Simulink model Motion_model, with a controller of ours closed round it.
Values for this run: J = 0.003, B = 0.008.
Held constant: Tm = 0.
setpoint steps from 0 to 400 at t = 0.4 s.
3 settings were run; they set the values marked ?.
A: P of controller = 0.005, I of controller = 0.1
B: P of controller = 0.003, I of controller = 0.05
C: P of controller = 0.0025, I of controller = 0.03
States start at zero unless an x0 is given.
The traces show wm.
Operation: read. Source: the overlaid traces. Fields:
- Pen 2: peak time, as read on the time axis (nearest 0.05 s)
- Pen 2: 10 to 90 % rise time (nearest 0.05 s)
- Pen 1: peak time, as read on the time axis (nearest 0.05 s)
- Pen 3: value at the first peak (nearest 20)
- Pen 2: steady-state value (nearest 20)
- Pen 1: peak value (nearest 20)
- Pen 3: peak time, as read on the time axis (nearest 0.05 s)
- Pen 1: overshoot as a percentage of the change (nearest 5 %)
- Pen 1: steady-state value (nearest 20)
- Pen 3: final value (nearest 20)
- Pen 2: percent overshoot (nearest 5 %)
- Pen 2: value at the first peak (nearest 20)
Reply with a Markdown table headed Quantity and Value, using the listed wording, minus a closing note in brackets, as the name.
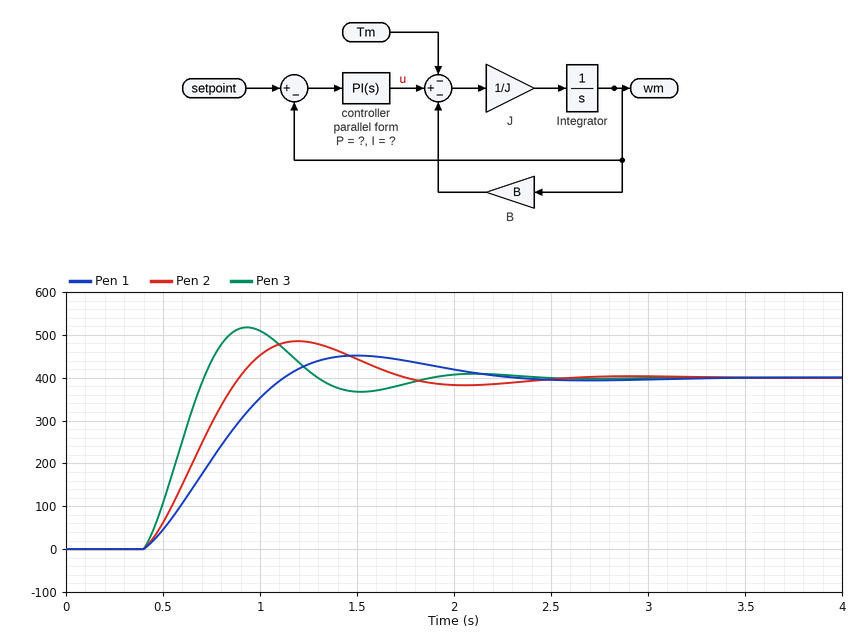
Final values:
| Quantity | Value |
|---|---|
| Pen 2: peak time, as read on the time axis | 1.20 s |
| Pen 2: 10 to 90 % rise time | 0.35 s |
| Pen 1: peak time, as read on the time axis | 1.50 s |
| Pen 3: value at the first peak | 520 |
| Pen 2: steady-state value | 400 |
| Pen 1: peak value | 460 |
| Pen 3: peak time, as read on the time axis | 0.95 s |
| Pen 1: overshoot as a percentage of the change | 15 % |
| Pen 1: steady-state value | 400 |
| Pen 3: final value | 400 |
| Pen 2: percent overshoot | 20 % |
| Pen 2: value at the first peak | 480 |
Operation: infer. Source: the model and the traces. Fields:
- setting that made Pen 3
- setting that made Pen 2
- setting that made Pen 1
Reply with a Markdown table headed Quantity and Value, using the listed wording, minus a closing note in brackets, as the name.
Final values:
| Quantity | Value |
|---|---|
| setting that made Pen 3 | A |
| setting that made Pen 2 | B |
| setting that made Pen 1 | C |
